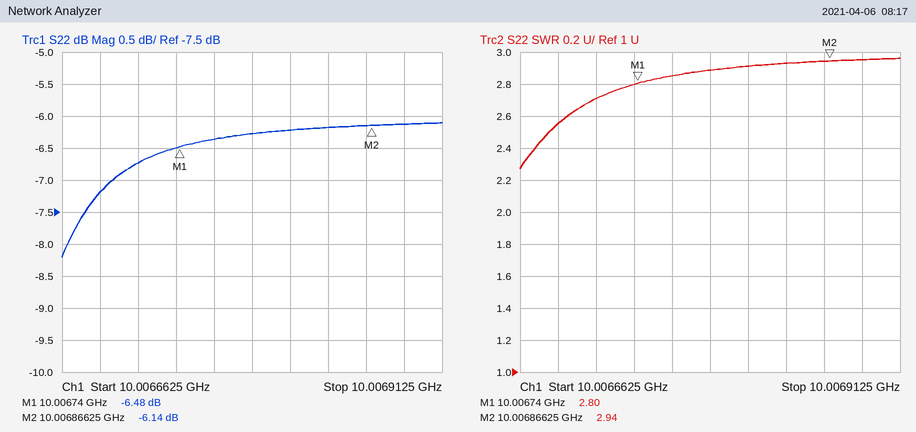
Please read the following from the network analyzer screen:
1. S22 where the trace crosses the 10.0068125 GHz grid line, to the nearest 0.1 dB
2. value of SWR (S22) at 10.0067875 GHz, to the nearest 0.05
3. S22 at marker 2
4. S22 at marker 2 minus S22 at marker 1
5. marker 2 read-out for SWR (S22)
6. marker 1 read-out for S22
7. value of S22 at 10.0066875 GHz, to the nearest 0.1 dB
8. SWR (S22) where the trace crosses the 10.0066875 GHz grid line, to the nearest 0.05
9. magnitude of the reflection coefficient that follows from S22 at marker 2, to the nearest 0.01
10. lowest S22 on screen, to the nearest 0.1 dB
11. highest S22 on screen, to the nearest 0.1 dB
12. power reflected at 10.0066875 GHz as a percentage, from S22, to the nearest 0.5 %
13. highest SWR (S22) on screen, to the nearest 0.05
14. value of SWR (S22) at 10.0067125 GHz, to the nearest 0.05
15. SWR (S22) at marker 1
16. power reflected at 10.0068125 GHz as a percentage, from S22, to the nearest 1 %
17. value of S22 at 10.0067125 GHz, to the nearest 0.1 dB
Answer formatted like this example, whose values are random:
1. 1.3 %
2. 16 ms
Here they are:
1. -6.2 dB
2. 2.90
3. -6.14 dB
4. 0.34 dB
5. 2.94
6. -6.48 dB
7. -7.2 dB
8. 2.55
9. 0.49
10. -8.2 dB
11. -6.1 dB
12. 19.0 %
13. 2.95
14. 2.70
15. 2.80
16. 24 %
17. -6.7 dB
